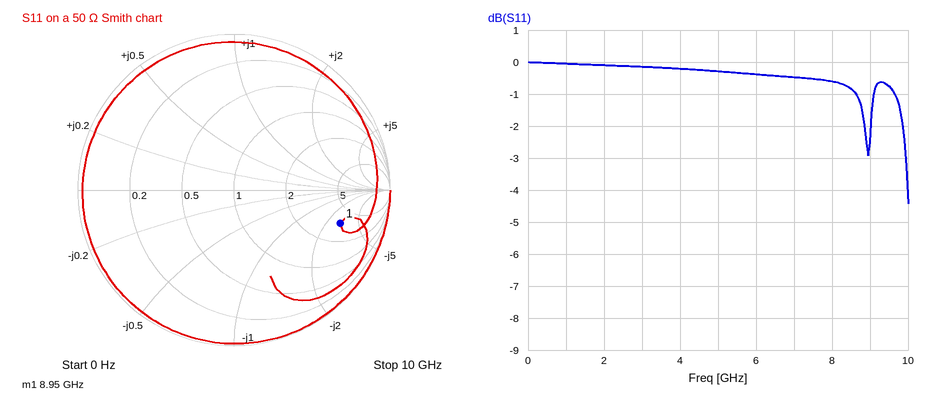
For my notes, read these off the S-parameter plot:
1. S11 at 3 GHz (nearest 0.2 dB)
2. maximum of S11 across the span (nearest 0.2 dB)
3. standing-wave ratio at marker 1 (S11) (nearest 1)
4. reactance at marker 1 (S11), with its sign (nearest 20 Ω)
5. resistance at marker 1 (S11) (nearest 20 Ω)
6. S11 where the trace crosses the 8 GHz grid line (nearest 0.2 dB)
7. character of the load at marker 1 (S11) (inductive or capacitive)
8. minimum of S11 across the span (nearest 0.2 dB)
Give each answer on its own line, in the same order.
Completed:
-0.2 dB
0.0 dB
6
-140 Ω
160 Ω
-0.6 dB
capacitive
-4.4 dB
